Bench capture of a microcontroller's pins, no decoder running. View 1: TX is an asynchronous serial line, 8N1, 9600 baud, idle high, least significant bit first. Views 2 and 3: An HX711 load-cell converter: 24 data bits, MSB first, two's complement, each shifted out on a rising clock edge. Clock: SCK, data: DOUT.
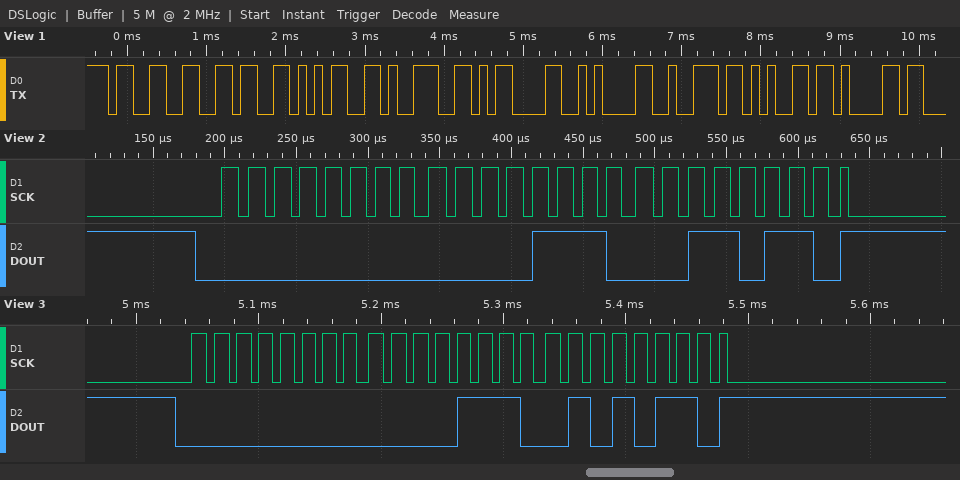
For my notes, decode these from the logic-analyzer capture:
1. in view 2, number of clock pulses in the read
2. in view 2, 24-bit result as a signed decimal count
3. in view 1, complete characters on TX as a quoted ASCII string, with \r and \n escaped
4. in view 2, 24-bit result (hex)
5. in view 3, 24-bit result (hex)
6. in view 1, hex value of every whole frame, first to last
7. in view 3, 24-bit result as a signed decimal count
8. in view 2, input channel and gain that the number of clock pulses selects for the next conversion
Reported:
25
3638
"3659\r\nrea"
0x000E36
0x000E56
33 36 35 39 0D 0A 72 65 61
3670
channel A, gain 128
